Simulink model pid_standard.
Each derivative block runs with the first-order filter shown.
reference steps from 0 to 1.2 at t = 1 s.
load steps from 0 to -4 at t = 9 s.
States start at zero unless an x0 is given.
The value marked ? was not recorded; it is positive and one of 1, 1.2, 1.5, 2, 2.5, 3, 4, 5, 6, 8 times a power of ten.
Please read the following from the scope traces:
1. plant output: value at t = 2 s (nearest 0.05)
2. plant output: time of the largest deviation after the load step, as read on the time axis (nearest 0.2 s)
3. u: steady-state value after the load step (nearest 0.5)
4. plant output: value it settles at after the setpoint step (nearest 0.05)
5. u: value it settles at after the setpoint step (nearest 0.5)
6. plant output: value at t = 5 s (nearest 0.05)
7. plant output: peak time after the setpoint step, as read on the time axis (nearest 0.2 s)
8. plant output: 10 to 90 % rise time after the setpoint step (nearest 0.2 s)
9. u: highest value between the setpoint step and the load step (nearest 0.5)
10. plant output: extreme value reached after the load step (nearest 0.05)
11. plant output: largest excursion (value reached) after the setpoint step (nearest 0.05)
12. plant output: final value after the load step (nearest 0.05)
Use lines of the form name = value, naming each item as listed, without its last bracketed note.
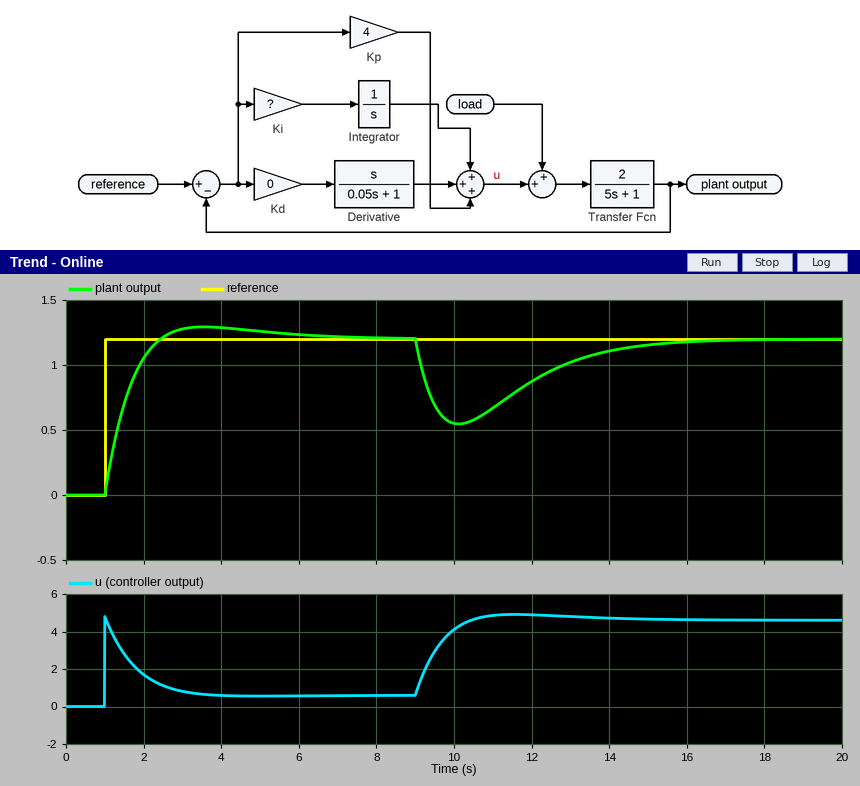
plant output: value at t = 2 s = 1.05
plant output: time of the largest deviation after the load step, as read on the time axis = 10.2 s
u: steady-state value after the load step = 4.5
plant output: value it settles at after the setpoint step = 1.20
u: value it settles at after the setpoint step = 0.5
plant output: value at t = 5 s = 1.25
plant output: peak time after the setpoint step, as read on the time axis = 3.6 s
plant output: 10 to 90 % rise time after the setpoint step = 1.0 s
u: highest value between the setpoint step and the load step = 5.0
plant output: extreme value reached after the load step = 0.55
plant output: largest excursion (value reached) after the setpoint step = 1.30
plant output: final value after the load step = 1.20
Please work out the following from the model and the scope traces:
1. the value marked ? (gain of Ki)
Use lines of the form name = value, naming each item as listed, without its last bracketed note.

the value marked ? = 2
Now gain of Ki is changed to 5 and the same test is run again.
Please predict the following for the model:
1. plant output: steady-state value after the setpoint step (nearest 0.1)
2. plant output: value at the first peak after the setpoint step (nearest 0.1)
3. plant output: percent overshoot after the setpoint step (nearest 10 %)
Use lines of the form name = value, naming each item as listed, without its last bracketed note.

plant output: steady-state value after the setpoint step = 1.2
plant output: value at the first peak after the setpoint step = 1.4
plant output: percent overshoot after the setpoint step = 20 %
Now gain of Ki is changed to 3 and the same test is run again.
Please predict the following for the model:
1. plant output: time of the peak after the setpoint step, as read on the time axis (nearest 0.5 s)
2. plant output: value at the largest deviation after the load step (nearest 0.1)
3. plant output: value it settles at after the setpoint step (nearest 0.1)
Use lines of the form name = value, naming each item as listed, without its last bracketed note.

plant output: time of the peak after the setpoint step, as read on the time axis = 3.0 s
plant output: value at the largest deviation after the load step = 0.6
plant output: value it settles at after the setpoint step = 1.2
